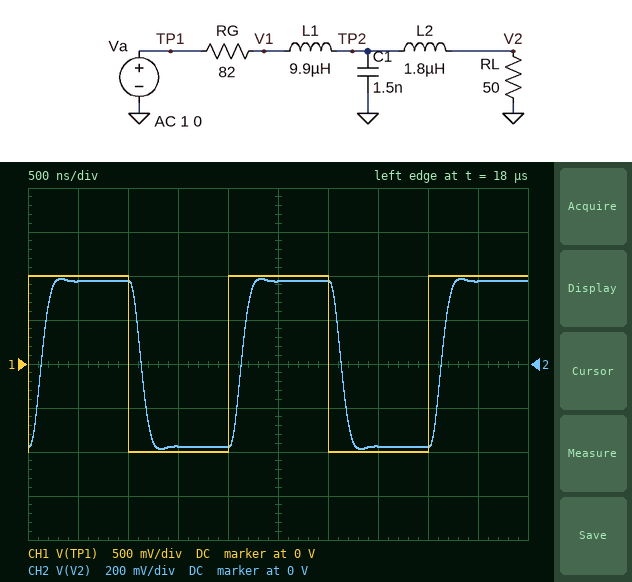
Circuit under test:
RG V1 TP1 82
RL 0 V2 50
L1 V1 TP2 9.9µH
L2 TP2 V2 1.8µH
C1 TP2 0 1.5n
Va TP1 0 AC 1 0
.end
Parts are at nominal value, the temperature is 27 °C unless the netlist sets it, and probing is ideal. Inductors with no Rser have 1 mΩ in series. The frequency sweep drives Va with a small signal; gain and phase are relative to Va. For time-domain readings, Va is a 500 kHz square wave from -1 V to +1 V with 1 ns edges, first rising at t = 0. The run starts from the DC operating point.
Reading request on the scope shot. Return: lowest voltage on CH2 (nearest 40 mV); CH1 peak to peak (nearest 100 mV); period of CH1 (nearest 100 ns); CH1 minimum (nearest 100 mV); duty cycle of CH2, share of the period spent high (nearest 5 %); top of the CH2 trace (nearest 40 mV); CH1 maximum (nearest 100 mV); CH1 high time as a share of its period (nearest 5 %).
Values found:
-400 mV
2.0 V
2.0 µs
-1.0 V
50 %
400 mV
1.0 V
50 %
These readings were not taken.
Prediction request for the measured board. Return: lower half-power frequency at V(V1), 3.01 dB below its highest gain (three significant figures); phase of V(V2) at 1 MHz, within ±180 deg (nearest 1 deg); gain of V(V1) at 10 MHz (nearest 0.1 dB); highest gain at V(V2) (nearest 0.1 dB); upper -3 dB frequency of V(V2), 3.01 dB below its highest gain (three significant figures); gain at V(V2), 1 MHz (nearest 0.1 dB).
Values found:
2.22 MHz
-48 deg
-0.1 dB
-8.4 dB
2.25 MHz
-9.0 dB
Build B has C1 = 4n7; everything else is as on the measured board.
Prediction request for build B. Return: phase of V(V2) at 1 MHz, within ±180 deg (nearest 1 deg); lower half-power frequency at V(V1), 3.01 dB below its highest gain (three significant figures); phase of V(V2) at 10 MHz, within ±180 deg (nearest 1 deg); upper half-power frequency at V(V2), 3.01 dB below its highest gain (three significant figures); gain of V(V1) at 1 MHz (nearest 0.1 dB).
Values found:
-86 deg
1.74 MHz
122 deg
1.10 MHz
-8.3 dB
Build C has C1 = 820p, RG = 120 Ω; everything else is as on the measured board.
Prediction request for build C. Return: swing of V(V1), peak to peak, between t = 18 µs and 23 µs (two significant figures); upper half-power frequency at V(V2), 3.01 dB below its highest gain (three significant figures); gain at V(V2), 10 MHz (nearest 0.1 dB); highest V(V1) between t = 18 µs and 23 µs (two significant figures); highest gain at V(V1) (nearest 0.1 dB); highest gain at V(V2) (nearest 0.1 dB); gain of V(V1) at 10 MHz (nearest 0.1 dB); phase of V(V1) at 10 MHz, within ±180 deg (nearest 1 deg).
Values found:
3.4 V
3.55 MHz
-36.5 dB
1.7 V
0 dB
-10.6 dB
-0.2 dB
11 deg
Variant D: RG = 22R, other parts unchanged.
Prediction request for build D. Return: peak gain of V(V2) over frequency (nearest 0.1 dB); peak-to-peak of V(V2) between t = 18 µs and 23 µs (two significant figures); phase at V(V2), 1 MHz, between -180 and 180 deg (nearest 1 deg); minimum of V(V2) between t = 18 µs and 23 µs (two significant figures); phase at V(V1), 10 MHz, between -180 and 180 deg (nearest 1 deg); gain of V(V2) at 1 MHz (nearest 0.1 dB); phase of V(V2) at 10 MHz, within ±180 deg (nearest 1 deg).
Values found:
-3.2 dB
1.4 V
-62 deg
-690 mV
2 deg
-4.8 dB
118 deg
